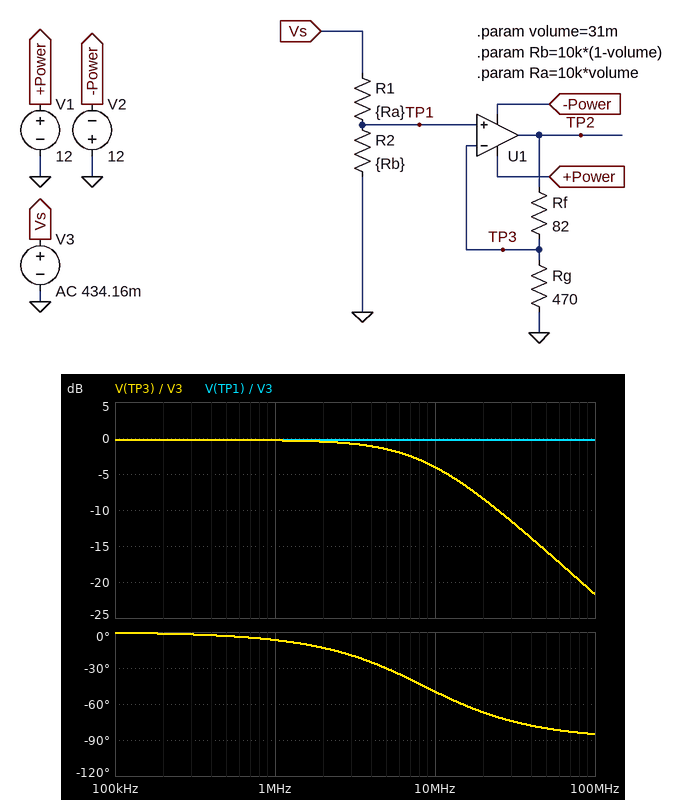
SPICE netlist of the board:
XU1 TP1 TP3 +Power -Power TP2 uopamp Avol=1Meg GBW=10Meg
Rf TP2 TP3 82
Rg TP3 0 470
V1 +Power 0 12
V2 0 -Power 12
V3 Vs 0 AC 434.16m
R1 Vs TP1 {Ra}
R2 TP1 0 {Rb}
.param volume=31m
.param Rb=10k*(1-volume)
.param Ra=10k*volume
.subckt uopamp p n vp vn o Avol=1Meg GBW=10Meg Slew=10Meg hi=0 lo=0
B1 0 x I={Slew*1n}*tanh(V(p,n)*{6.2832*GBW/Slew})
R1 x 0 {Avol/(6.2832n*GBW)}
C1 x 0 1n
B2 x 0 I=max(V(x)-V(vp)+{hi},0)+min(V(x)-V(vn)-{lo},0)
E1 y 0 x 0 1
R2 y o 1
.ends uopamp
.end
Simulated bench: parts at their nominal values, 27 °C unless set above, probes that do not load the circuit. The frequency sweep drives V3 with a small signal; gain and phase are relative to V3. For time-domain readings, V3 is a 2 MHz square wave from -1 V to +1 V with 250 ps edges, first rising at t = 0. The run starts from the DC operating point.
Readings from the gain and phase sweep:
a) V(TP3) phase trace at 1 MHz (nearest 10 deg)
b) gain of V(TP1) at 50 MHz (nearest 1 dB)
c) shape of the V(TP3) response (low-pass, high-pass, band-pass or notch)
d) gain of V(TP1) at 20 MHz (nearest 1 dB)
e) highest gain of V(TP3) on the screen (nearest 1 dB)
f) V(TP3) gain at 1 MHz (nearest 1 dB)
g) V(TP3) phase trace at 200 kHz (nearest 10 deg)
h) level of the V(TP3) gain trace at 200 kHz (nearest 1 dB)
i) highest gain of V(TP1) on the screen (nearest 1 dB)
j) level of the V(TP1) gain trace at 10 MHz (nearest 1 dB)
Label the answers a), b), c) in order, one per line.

a) -10 deg
b) 0 dB
c) low-pass
d) 0 dB
e) 0 dB
f) 0 dB
g) 0 deg
h) 0 dB
i) 0 dB
j) 0 dB
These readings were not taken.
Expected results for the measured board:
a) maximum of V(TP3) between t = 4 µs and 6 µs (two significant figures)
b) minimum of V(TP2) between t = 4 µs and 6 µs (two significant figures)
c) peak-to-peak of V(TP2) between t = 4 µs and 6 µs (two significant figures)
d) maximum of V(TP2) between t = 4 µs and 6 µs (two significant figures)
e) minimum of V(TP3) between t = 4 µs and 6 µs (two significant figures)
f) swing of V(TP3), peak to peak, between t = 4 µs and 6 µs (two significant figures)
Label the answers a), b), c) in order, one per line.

a) 950 mV
b) -1.1 V
c) 2.2 V
d) 1.1 V
e) -950 mV
f) 1.9 V
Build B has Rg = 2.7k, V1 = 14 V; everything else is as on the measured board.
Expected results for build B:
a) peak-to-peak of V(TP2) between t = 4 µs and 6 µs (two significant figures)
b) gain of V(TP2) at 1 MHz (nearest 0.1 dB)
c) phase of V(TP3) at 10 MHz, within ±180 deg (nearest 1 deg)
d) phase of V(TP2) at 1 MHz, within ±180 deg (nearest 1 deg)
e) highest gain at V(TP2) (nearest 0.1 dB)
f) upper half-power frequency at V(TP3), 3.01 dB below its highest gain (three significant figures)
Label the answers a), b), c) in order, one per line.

a) 2.0 V
b) -0.1 dB
c) -46 deg
d) -6 deg
e) 0 dB
f) 9.70 MHz
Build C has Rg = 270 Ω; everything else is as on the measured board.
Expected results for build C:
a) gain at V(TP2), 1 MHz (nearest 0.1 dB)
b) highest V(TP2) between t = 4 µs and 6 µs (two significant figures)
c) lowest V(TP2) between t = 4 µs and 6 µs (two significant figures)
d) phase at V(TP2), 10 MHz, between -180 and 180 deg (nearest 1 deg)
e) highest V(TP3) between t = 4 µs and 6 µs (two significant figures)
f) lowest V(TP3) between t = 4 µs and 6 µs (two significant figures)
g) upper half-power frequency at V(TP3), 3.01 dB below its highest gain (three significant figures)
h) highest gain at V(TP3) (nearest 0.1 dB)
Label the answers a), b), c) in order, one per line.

a) 2.0 dB
b) 1.2 V
c) -1.2 V
d) -53 deg
e) 910 mV
f) -910 mV
g) 7.65 MHz
h) -0.3 dB
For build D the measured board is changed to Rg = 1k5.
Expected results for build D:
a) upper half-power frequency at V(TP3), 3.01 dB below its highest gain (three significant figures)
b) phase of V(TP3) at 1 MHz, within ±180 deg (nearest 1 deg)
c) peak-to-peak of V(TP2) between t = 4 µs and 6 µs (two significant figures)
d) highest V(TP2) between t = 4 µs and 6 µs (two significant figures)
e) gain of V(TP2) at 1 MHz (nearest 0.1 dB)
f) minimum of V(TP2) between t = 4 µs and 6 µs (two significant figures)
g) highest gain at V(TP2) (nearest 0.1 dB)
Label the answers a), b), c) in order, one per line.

a) 9.48 MHz
b) -6 deg
c) 2.0 V
d) 1.0 V
e) 0.1 dB
f) -1.0 V
g) 0.2 dB
